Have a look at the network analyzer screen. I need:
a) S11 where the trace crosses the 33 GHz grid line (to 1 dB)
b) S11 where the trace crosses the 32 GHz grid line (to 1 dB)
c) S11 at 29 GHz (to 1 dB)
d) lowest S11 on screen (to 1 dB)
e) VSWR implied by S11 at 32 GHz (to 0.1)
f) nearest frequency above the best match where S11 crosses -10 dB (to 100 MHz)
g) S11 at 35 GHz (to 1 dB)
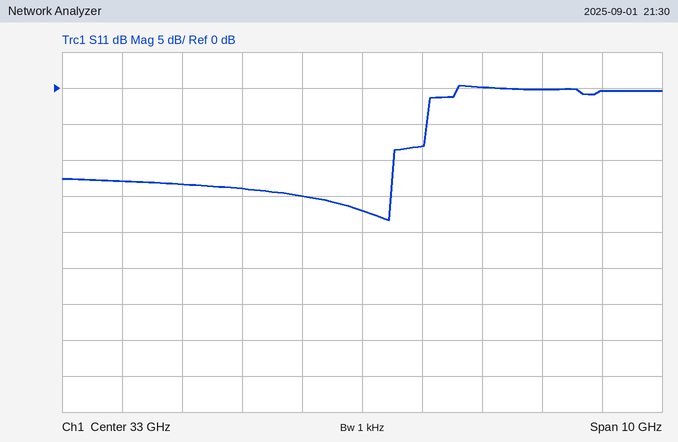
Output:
-17 dB
-15 dB
-13 dB
-18 dB
1.4
33.5 GHz
0 dB
